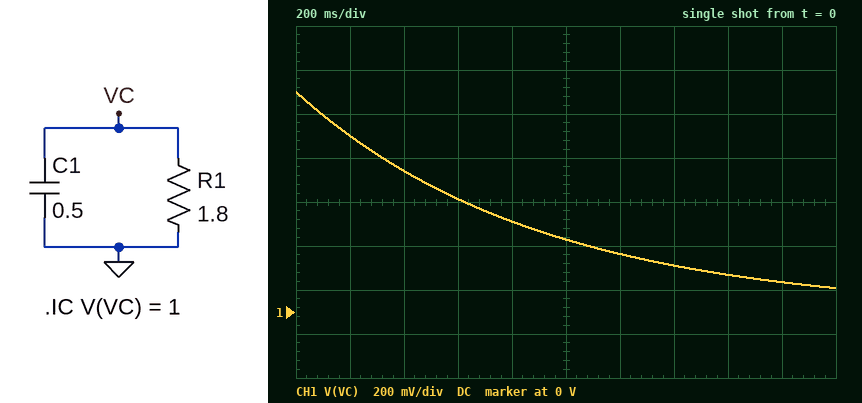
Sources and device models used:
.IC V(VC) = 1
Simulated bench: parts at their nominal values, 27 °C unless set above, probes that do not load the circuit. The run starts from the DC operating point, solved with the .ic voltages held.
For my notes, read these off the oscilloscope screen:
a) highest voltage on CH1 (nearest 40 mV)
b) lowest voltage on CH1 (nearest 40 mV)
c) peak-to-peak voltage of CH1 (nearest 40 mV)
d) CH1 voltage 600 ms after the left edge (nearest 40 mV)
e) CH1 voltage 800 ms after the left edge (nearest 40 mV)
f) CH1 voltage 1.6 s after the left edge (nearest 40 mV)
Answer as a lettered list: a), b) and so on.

a) 1.00 V
b) 120 mV
c) 880 mV
d) 520 mV
e) 400 mV
f) 160 mV
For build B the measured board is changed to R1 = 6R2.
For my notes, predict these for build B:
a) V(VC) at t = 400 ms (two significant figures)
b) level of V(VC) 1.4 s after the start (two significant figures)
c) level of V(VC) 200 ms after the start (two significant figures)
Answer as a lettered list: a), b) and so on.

a) 880 mV
b) 640 mV
c) 940 mV
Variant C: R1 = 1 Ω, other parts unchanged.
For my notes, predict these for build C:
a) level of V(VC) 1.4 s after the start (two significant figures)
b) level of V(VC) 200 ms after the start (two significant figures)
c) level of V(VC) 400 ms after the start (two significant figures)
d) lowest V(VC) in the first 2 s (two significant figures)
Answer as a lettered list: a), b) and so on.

a) 61 mV
b) 670 mV
c) 450 mV
d) 18 mV
